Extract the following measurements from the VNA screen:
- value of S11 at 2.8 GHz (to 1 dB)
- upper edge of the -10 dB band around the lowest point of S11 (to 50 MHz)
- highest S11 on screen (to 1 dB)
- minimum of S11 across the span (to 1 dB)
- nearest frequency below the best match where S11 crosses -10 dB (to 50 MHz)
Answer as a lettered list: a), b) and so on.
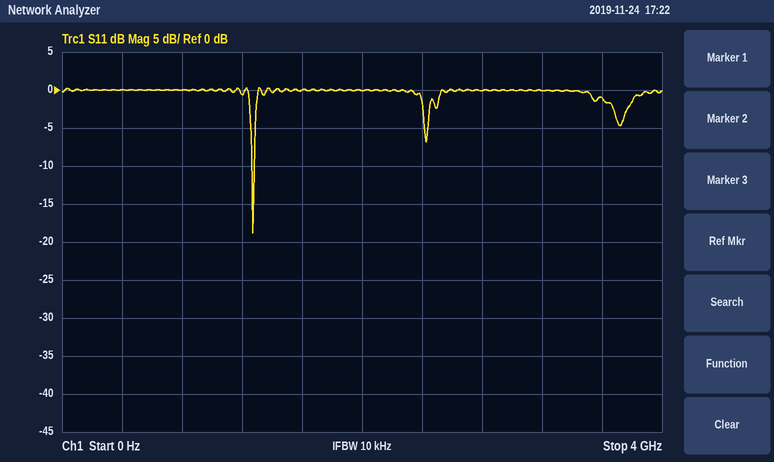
a) 0 dB
b) 1.30 GHz
c) 0 dB
d) -19 dB
e) 1.25 GHz
